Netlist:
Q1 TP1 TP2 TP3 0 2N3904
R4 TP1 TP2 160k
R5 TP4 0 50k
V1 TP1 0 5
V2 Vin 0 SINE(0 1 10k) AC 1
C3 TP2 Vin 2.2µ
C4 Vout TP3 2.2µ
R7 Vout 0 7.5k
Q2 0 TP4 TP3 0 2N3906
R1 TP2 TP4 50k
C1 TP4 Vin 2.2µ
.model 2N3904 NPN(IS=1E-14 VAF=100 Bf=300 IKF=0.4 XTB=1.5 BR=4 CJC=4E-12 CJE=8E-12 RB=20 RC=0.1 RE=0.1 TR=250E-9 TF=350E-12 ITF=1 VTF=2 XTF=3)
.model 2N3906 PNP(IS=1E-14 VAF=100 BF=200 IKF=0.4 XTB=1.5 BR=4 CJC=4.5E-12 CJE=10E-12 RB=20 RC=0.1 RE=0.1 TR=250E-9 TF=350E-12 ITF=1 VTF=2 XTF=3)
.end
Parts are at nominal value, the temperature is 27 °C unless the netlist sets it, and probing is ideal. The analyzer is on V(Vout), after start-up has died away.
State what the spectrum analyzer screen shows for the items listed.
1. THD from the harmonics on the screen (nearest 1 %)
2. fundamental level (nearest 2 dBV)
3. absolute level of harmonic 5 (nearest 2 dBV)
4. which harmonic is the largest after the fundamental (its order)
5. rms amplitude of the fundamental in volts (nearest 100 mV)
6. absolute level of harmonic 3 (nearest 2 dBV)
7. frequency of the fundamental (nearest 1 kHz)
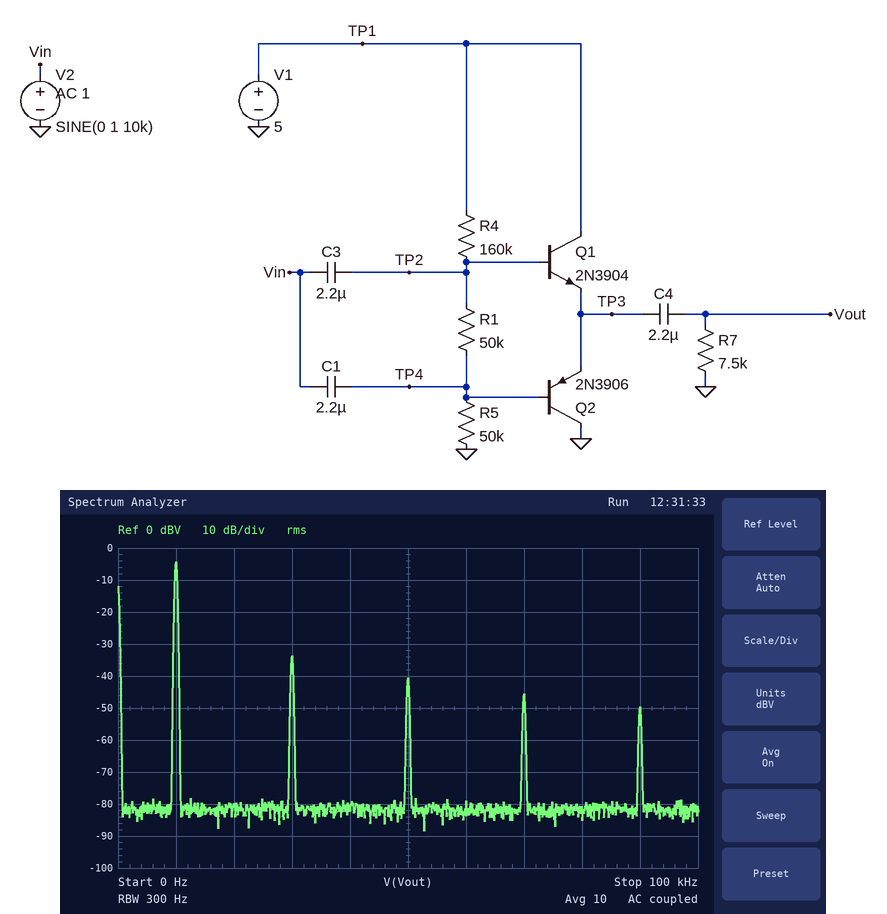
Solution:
4 %
-4 dBV
-40 dBV
3
600 mV
-34 dBV
10 kHz
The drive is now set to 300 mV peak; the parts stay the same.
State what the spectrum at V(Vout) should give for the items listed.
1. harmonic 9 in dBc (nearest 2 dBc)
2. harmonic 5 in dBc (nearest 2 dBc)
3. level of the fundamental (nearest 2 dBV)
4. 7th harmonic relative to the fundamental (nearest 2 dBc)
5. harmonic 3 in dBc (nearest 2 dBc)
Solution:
-50 dBc
-34 dBc
-16 dBV
-42 dBc
-24 dBc
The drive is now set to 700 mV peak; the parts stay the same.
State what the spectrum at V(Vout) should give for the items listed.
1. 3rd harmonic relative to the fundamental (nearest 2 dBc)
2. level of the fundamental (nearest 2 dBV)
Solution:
-28 dBc
-8 dBV
